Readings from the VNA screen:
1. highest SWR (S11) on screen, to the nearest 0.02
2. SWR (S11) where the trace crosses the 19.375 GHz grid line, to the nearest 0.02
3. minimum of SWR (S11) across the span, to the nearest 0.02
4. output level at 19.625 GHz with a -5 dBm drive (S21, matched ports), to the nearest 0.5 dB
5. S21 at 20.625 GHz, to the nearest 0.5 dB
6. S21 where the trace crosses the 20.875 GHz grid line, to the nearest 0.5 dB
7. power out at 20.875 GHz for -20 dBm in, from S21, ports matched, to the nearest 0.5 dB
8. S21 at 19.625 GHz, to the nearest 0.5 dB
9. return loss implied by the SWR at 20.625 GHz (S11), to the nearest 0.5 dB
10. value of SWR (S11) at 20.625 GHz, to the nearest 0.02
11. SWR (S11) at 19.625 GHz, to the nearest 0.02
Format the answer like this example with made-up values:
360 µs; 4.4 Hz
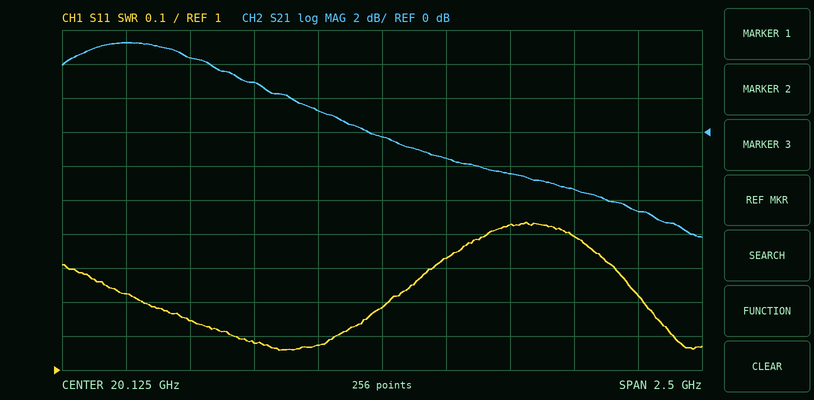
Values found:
1.44; 1.14; 1.06; -2.0 dBm; -2.5 dB; -3.5 dB; -23.5 dBm; 3.0 dB; 15.0 dB; 1.42; 1.08
